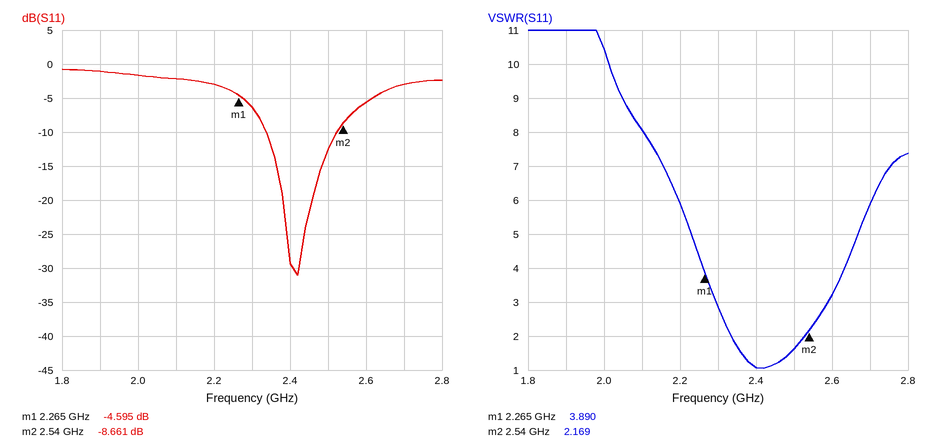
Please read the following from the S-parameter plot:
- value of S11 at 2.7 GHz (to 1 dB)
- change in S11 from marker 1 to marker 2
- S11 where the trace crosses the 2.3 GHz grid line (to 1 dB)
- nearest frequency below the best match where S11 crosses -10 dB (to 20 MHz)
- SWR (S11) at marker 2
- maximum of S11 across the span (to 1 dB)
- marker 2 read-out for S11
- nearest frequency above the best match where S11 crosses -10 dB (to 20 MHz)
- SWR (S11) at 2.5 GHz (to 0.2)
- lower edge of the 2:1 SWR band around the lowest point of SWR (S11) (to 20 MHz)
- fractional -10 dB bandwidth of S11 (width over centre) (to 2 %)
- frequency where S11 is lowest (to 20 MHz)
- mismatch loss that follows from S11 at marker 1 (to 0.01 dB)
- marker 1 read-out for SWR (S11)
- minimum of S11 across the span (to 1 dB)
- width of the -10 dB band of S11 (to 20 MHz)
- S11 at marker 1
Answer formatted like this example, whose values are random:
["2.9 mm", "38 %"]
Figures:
["-3 dB", "-4.066 dB", "-6 dB", "2.34 GHz", "2.169", "-1 dB", "-8.661 dB", "2.52 GHz", "1.6", "2.34 GHz", "8 %", "2.42 GHz", "1.85 dB", "3.890", "-31 dB", "180 MHz", "-4.595 dB"]
